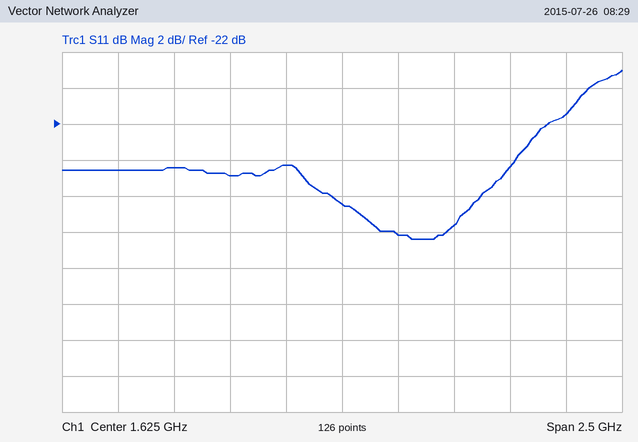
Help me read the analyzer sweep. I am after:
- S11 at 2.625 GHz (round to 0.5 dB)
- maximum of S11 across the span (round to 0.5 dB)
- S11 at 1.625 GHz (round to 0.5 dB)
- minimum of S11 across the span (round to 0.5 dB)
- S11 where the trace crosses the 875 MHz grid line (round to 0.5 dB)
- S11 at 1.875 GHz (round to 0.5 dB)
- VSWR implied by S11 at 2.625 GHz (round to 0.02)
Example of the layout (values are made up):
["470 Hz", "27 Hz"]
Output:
["-21.5 dB", "-19.0 dB", "-26.5 dB", "-28.5 dB", "-24.5 dB", "-28.0 dB", "1.18"]
